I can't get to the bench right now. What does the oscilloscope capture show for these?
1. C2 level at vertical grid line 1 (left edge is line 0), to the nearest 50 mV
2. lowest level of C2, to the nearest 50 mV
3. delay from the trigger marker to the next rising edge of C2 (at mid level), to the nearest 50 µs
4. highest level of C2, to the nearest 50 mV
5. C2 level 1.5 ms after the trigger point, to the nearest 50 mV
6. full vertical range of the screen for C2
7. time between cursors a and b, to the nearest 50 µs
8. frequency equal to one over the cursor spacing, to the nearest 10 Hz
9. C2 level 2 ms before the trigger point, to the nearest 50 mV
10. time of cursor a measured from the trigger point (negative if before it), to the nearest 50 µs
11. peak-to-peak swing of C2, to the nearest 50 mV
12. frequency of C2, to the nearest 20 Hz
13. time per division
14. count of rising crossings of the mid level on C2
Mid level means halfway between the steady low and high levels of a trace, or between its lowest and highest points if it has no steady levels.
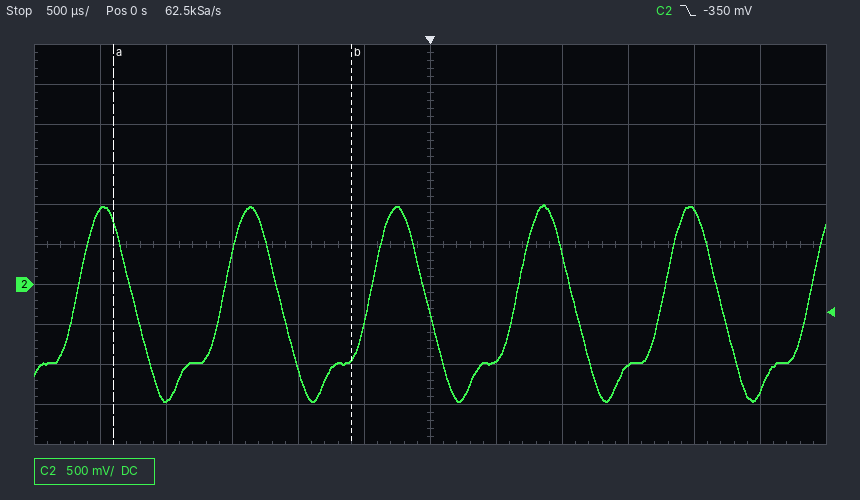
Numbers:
950 mV
-1.45 V
650 µs
1.00 V
-1.00 V
5 V
1.80 ms
560 Hz
-1.45 V
-2.40 ms
2.45 V
900 Hz
500 µs
6
